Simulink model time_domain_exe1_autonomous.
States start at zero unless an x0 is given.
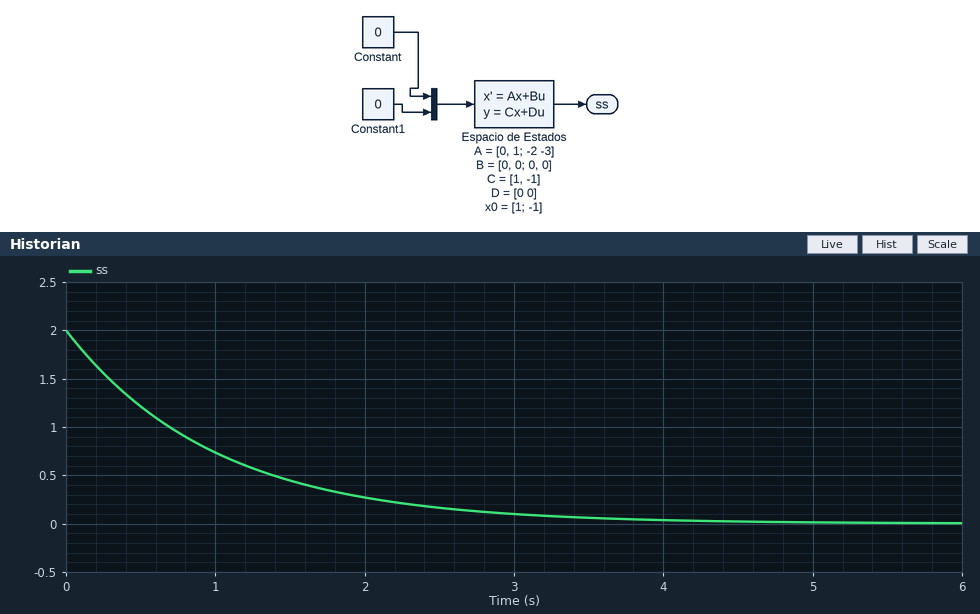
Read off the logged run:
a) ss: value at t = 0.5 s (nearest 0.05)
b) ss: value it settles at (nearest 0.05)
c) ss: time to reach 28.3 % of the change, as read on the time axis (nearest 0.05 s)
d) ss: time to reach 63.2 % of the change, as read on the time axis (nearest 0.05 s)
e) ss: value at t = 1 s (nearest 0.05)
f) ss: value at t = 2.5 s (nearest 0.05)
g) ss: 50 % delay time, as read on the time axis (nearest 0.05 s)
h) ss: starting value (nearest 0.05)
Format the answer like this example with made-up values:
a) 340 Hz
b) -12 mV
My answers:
a) 1.20
b) 0.00
c) 0.35 s
d) 1.00 s
e) 0.75
f) 0.15
g) 0.70 s
h) 2.00
